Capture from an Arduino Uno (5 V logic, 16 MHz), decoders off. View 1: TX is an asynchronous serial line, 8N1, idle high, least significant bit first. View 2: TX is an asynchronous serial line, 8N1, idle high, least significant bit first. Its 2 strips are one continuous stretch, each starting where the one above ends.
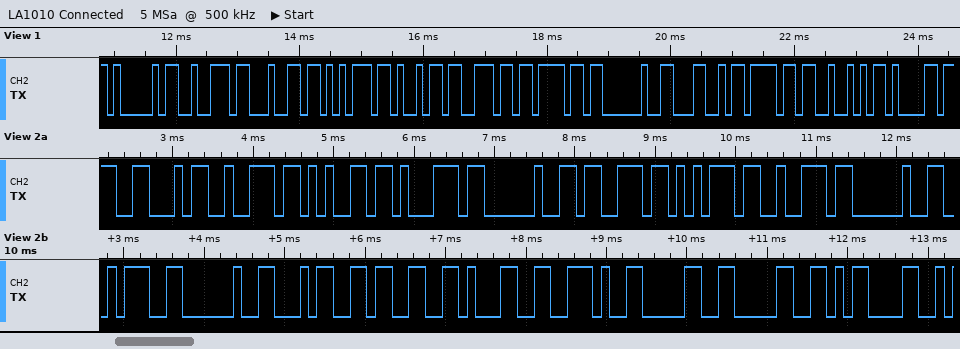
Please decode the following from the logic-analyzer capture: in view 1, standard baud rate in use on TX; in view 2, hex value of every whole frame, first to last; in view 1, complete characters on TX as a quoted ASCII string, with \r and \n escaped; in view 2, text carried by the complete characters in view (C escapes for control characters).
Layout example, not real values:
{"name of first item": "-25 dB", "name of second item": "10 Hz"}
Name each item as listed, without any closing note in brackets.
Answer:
{"in view 1, standard baud rate in use on TX": "9600 baud", "in view 2, hex value of every whole frame, first to last": "46 72 65 71 20 73 75 72 20 3A 20 34 33 31 2E 30 30 0D", "in view 1, complete characters on TX as a quoted ASCII string, with \\r and \\n escaped": "\"Arduino LoRa\"", "in view 2, text carried by the complete characters in view": "\"Freq sur : 431.00\\r\""}
